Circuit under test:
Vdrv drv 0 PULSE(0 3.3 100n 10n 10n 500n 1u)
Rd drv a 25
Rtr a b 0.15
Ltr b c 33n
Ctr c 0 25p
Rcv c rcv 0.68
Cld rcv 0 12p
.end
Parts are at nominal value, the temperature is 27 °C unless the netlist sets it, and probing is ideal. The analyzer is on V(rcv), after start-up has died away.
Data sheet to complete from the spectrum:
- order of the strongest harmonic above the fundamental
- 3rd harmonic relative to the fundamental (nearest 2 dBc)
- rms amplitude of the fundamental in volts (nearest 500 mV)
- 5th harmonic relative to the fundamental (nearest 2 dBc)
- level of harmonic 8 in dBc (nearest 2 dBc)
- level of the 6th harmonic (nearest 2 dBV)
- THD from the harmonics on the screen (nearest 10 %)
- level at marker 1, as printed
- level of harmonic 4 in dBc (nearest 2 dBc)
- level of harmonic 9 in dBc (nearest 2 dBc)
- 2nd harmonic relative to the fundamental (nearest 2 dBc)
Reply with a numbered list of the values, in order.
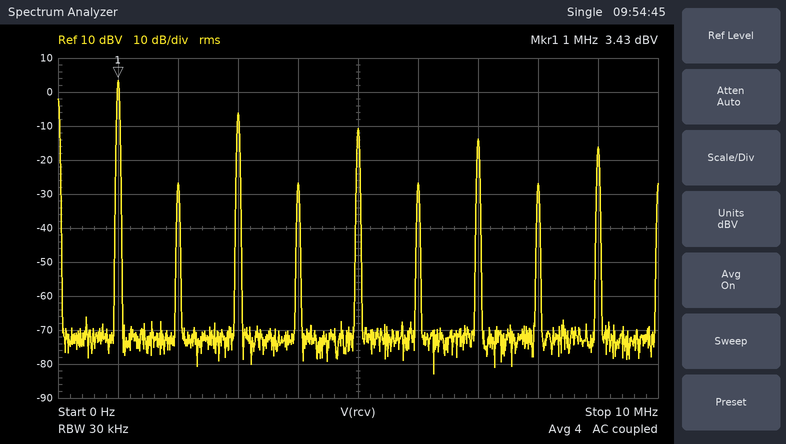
1. 3
2. -10 dBc
3. 1.5 V
4. -14 dBc
5. -30 dBc
6. -26 dBV
7. 40 %
8. 3.43 dBV
9. -30 dBc
10. -20 dBc
11. -30 dBc
